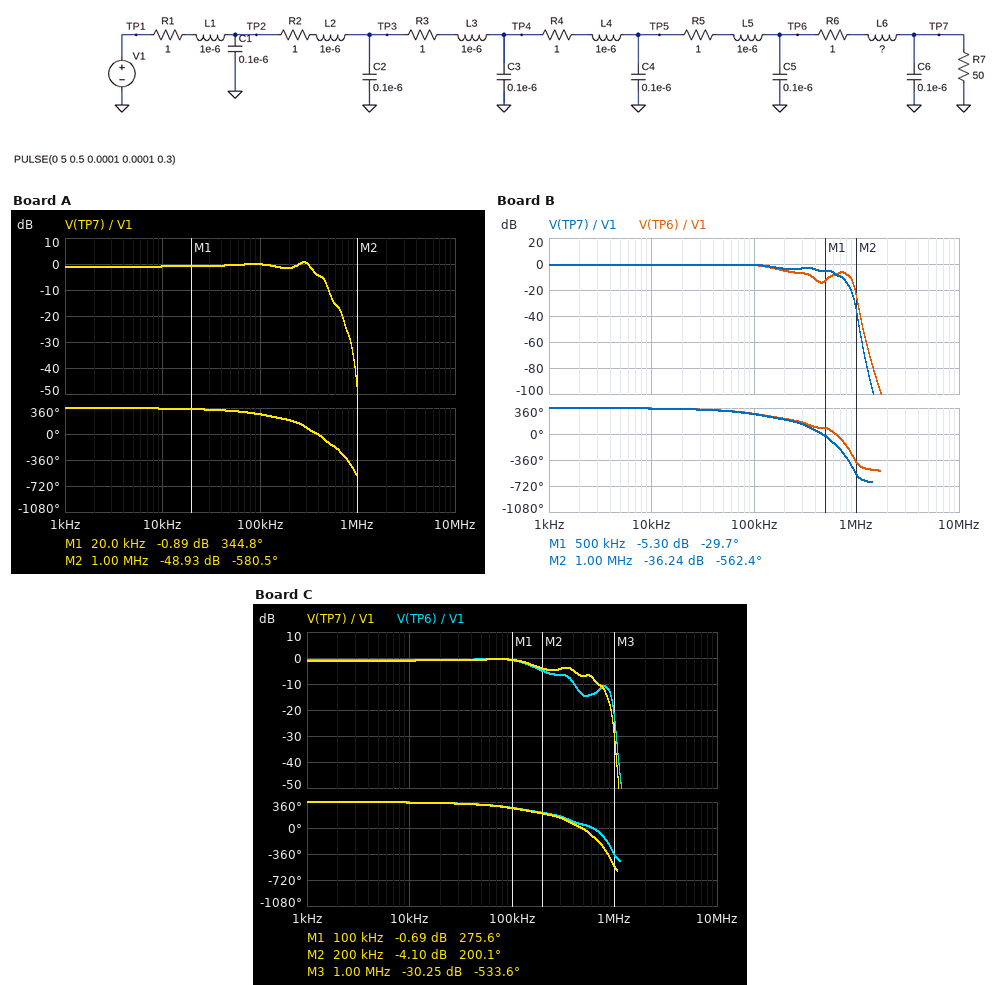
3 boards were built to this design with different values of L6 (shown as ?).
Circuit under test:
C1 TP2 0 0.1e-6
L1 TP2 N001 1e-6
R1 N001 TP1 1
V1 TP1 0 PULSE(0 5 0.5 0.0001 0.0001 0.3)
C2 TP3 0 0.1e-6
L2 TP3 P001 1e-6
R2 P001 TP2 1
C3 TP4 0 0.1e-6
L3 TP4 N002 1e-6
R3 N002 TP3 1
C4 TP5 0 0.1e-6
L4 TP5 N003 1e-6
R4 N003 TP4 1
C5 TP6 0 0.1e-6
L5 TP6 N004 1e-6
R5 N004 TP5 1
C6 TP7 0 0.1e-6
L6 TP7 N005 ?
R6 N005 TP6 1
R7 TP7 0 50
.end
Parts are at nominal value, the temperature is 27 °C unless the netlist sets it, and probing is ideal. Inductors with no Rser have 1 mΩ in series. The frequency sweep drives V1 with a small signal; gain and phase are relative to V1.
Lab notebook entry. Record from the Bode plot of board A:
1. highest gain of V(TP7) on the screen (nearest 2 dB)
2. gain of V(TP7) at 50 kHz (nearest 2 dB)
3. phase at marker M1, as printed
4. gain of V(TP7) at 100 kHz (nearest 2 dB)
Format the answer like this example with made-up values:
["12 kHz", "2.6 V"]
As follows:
["0 dB", "0 dB", "344.8 deg", "0 dB"]
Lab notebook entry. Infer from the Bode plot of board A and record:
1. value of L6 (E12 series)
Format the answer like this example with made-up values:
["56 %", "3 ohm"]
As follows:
["3.3 µH"]
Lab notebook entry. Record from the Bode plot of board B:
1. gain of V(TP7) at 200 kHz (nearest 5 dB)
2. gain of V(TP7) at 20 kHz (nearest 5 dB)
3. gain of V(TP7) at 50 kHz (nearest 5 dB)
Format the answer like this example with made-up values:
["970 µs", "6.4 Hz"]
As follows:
["-5 dB", "0 dB", "0 dB"]
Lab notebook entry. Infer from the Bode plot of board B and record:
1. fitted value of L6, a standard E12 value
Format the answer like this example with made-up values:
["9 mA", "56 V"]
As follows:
["1.2 µH"]
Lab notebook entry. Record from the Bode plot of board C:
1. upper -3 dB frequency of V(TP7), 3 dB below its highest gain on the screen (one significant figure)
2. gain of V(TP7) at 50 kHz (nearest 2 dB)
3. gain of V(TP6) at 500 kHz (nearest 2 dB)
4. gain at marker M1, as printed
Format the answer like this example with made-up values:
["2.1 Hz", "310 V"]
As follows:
["200 kHz", "0 dB", "-14 dB", "-0.69 dB"]
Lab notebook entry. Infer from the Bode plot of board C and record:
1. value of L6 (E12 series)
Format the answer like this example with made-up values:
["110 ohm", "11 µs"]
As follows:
["820 nH"]
